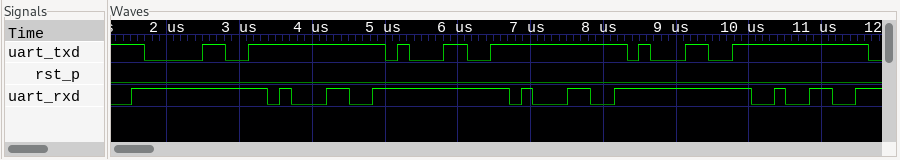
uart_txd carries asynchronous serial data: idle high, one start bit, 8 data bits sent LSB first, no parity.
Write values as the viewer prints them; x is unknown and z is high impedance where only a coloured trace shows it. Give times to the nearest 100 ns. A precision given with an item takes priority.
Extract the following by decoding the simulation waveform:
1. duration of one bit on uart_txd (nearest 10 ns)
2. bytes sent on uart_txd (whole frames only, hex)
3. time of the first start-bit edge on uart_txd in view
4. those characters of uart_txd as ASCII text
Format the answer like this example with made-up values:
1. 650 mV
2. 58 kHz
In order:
1. 160 ns
2. 30, 31, 31
3. 1700 ns
4. "011"
